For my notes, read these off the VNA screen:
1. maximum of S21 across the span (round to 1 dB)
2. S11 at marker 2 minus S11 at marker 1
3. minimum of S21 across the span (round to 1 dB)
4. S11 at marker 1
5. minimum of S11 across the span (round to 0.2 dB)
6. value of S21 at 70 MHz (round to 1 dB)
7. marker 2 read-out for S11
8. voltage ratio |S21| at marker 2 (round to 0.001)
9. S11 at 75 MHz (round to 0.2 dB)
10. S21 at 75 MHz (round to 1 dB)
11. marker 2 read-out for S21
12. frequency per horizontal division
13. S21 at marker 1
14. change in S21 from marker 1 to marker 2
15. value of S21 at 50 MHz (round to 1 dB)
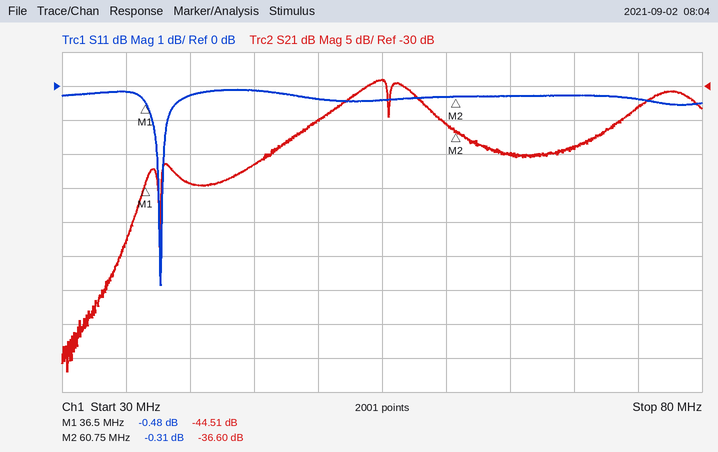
-29 dB
0.17 dB
-72 dB
-0.48 dB
-5.8 dB
-39 dB
-0.31 dB
0.015
-0.4 dB
-33 dB
-36.60 dB
5 MHz
-44.51 dB
7.91 dB
-35 dB
